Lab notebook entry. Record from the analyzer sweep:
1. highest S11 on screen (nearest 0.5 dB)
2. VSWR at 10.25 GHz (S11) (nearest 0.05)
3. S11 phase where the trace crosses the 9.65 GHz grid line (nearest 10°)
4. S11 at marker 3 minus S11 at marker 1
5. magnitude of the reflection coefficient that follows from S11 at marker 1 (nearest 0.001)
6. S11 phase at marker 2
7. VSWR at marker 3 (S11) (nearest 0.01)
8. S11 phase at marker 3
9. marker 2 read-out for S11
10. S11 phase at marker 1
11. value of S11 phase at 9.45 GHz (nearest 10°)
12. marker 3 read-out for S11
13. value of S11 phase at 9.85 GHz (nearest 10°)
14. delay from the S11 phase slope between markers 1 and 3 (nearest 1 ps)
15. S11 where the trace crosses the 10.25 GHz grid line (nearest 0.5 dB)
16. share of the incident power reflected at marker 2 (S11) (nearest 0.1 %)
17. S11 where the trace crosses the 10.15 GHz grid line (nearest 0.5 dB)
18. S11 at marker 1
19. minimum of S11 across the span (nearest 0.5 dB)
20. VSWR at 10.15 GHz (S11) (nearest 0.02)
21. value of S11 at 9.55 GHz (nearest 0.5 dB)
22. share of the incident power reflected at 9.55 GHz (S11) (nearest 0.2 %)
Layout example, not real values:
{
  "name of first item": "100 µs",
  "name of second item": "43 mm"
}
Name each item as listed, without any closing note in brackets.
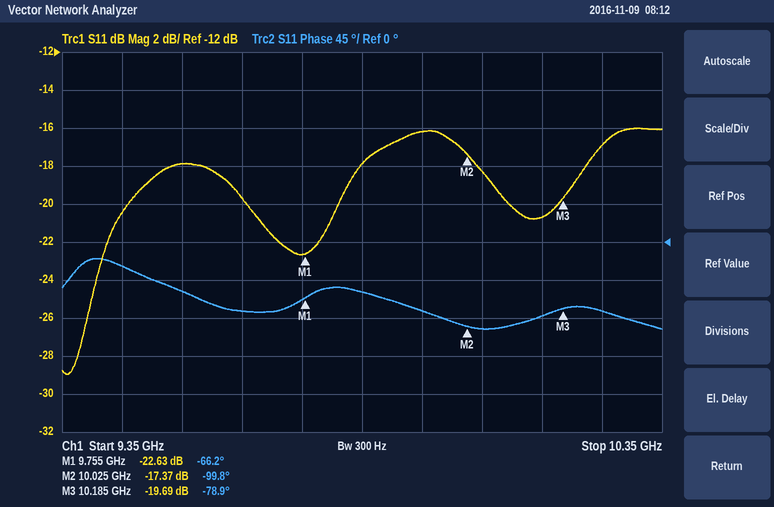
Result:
{
  "highest S11 on screen": "-16.0 dB",
  "VSWR at 10.25 GHz (S11)": "1.35",
  "S11 phase where the trace crosses the 9.65 GHz grid line": "-80°",
  "S11 at marker 3 minus S11 at marker 1": "2.94 dB",
  "magnitude of the reflection coefficient that follows from S11 at marker 1": "0.074",
  "S11 phase at marker 2": "-99.8°",
  "VSWR at marker 3 (S11)": "1.23",
  "S11 phase at marker 3": "-78.9°",
  "marker 2 read-out for S11": "-17.37 dB",
  "S11 phase at marker 1": "-66.2°",
  "value of S11 phase at 9.45 GHz": "-30°",
  "marker 3 read-out for S11": "-19.69 dB",
  "value of S11 phase at 9.85 GHz": "-60°",
  "delay from the S11 phase slope between markers 1 and 3": "82 ps",
  "S11 where the trace crosses the 10.25 GHz grid line": "-17.0 dB",
  "share of the incident power reflected at marker 2 (S11)": "1.8 %",
  "S11 where the trace crosses the 10.15 GHz grid line": "-20.5 dB",
  "S11 at marker 1": "-22.63 dB",
  "minimum of S11 across the span": "-29.0 dB",
  "VSWR at 10.15 GHz (S11)": "1.20",
  "value of S11 at 9.55 GHz": "-18.0 dB",
  "share of the incident power reflected at 9.55 GHz (S11)": "1.6 %"
}
